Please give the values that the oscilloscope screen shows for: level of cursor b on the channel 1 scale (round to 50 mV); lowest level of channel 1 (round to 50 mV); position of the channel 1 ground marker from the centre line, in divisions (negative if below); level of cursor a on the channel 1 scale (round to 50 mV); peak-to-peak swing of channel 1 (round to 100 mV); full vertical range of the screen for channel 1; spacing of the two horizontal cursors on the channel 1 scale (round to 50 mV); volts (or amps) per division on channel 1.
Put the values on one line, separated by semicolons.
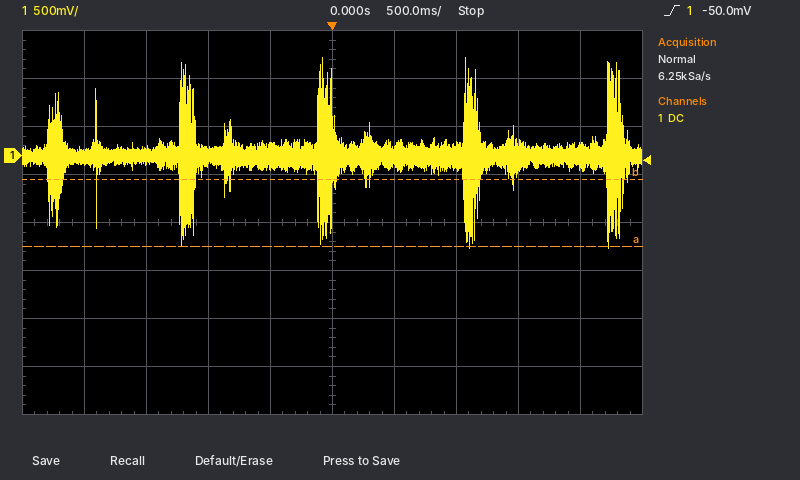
-250 mV; -950 mV; +1.4 div; -950 mV; 2.00 V; 4 V; 700 mV; 500 mV
